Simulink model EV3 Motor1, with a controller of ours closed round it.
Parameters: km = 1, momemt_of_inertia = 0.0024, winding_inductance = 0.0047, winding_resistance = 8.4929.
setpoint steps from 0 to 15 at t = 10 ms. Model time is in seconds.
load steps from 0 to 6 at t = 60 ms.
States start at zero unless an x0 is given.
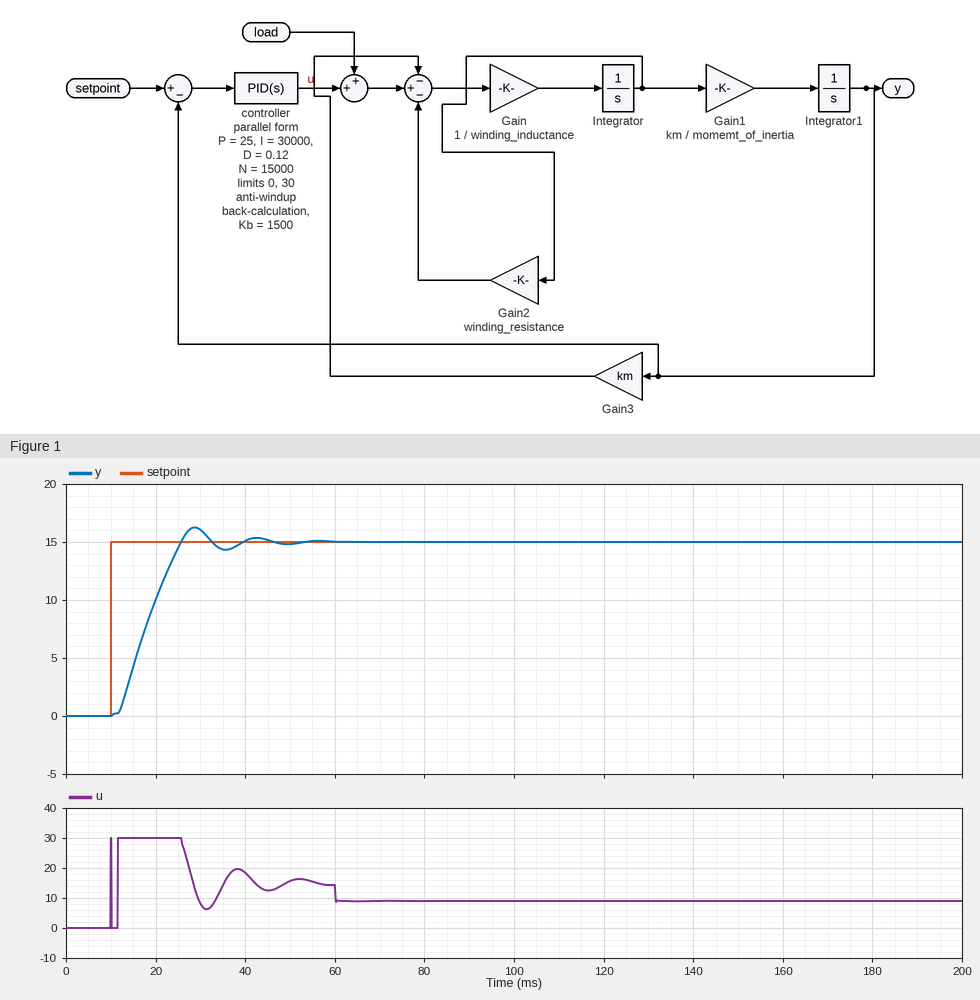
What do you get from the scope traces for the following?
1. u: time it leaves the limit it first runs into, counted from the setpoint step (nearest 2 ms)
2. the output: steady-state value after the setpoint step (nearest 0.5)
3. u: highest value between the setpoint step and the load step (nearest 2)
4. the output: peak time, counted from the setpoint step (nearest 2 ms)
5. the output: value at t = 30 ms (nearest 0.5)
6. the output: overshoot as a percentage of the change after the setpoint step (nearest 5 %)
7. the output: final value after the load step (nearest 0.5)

16 ms
15.0
30
18 ms
16.0
10 %
15.0
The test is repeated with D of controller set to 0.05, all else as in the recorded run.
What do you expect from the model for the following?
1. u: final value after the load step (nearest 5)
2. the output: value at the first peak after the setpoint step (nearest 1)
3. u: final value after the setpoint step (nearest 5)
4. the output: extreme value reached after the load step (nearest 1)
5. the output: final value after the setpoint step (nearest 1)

10
16
15
15
15
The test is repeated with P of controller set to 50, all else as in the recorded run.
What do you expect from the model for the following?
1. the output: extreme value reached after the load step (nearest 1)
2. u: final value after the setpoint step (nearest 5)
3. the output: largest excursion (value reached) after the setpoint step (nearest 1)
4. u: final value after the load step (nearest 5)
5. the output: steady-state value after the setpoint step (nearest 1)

15
15
16
10
15
